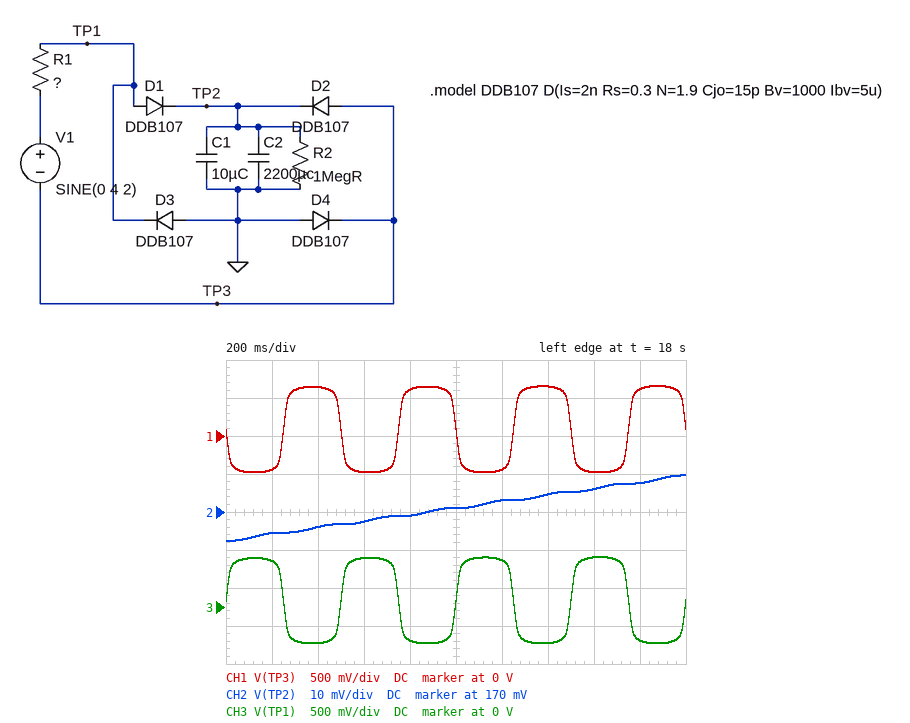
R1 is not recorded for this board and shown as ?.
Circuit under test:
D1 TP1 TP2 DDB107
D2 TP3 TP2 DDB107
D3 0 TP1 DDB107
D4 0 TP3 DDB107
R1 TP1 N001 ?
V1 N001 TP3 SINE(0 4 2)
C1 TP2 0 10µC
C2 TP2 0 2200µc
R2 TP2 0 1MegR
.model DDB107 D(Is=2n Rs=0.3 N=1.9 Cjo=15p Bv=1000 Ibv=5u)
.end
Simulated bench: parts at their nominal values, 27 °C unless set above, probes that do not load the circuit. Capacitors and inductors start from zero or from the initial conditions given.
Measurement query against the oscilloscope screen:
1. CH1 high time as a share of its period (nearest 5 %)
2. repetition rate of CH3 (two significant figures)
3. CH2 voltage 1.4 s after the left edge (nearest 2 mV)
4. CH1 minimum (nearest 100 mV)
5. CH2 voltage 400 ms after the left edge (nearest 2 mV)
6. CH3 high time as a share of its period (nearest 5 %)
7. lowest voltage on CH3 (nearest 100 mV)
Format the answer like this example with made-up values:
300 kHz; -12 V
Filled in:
50 %; 2.0 Hz; 174 mV; -500 mV; 166 mV; 50 %; -500 mV
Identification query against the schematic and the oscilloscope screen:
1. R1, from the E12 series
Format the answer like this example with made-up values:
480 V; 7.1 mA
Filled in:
82 kΩ
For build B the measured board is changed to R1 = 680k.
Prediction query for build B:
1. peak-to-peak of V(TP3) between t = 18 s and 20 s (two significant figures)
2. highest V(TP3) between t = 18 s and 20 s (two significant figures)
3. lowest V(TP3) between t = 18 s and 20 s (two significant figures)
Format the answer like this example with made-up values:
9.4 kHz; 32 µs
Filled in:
790 mV; 410 mV; -380 mV
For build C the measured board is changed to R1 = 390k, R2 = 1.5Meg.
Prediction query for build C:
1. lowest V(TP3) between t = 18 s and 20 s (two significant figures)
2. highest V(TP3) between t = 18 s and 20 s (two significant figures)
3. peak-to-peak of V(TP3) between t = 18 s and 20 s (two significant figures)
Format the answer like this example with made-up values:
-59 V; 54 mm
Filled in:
-410 mV; 450 mV; 860 mV
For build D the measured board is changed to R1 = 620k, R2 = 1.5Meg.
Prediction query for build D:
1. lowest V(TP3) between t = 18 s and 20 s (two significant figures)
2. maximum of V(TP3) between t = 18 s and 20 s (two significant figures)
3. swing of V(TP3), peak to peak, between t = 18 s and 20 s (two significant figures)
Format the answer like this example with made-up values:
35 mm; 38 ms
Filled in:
-390 mV; 410 mV; 800 mV
